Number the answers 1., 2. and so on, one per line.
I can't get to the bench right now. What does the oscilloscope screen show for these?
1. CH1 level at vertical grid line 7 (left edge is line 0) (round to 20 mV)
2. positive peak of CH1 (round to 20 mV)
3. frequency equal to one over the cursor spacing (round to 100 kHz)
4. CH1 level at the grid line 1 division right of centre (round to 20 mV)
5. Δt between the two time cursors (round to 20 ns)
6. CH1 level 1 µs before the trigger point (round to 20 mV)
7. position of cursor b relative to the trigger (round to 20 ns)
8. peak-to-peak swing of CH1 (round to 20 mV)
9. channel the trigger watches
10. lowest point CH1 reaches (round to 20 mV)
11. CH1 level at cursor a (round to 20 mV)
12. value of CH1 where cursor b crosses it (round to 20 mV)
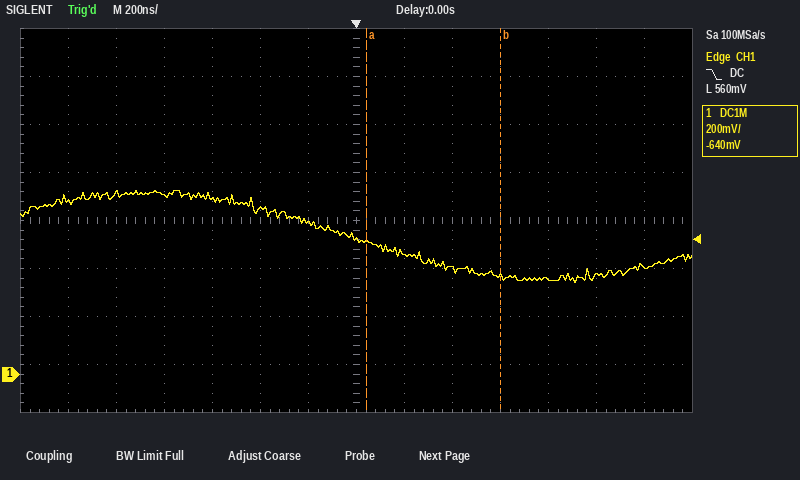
1. 560 mV
2. 760 mV
3. 1.8 MHz
4. 500 mV
5. 560 ns
6. 760 mV
7. +600 ns
8. 380 mV
9. CH1
10. 380 mV
11. 560 mV
12. 400 mV
